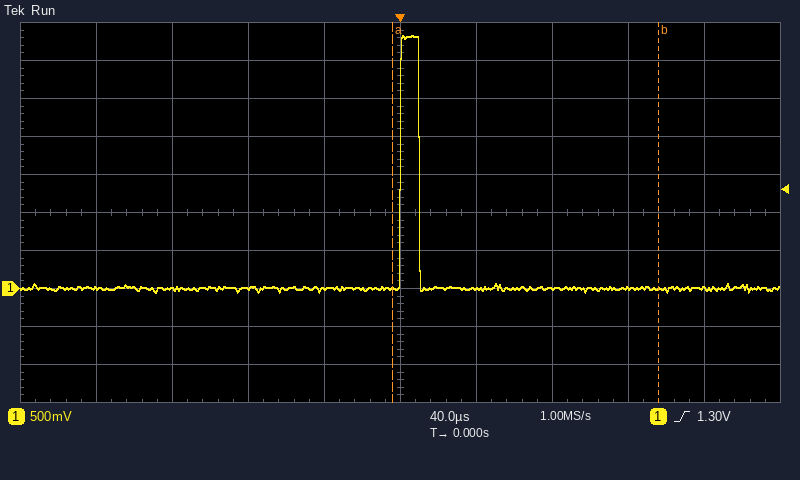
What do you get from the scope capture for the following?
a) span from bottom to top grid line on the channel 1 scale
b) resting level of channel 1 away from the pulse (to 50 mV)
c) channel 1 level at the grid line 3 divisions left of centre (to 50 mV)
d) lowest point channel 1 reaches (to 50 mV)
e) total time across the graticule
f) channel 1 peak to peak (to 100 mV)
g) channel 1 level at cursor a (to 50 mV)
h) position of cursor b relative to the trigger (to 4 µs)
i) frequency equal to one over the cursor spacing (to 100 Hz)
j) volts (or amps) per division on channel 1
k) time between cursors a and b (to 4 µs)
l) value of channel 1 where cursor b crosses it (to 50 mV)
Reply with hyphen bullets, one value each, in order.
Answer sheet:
- 5 V
- 0 mV
- 0 mV
- -50 mV
- 400 µs
- 3.40 V
- 0 mV
- +136 µs
- 7.1 kHz
- 500 mV
- 140 µs
- 0 mV
